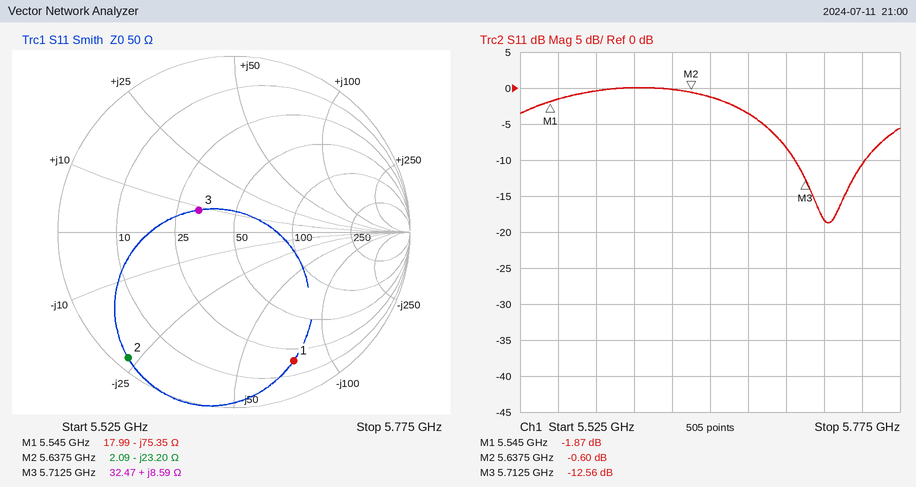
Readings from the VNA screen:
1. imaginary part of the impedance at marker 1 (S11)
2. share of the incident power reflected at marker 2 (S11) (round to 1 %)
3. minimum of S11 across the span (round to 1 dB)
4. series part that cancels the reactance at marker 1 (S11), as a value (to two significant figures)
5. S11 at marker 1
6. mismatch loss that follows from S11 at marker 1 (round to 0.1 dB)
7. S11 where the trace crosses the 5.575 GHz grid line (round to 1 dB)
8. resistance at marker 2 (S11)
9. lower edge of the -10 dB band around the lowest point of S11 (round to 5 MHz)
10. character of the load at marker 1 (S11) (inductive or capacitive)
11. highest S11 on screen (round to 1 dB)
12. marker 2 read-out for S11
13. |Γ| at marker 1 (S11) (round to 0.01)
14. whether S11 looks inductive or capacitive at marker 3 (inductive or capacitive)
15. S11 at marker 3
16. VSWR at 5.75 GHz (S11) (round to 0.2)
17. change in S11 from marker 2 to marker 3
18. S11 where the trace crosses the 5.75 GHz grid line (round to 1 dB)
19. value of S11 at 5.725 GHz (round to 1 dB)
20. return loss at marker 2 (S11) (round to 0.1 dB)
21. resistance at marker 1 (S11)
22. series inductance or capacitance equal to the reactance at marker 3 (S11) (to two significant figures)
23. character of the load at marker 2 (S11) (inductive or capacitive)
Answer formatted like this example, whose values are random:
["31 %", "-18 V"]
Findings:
["-75.35 Ω", "87 %", "-19 dB", "2.2 nH", "-1.87 dB", "4.6 dB", "0 dB", "2.09 Ω", "5.705 GHz", "capacitive", "0 dB", "-0.60 dB", "0.81", "inductive", "-12.56 dB", "1.8", "-11.96 dB", "-11 dB", "-18 dB", "0.6 dB", "17.99 Ω", "240 pH", "capacitive"]
